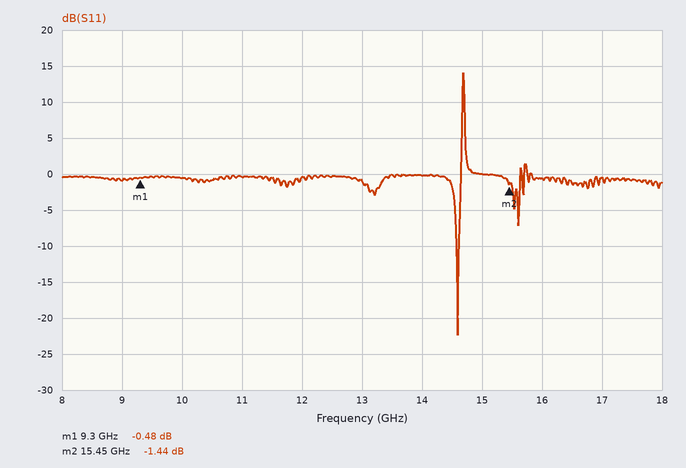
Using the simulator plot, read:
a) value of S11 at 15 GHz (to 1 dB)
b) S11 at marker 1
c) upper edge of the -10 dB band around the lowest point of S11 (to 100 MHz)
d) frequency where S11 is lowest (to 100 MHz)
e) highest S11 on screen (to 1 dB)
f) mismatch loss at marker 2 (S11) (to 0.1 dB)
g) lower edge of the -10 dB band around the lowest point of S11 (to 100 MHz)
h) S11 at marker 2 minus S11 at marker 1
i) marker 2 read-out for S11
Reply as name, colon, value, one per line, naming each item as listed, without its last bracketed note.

value of S11 at 15 GHz: 0 dB
S11 at marker 1: -0.48 dB
upper edge of the -10 dB band around the lowest point of S11: 14.6 GHz
frequency where S11 is lowest: 14.6 GHz
highest S11 on screen: 14 dB
mismatch loss at marker 2 (S11): 5.5 dB
lower edge of the -10 dB band around the lowest point of S11: 14.6 GHz
S11 at marker 2 minus S11 at marker 1: -0.96 dB
marker 2 read-out for S11: -1.44 dB
